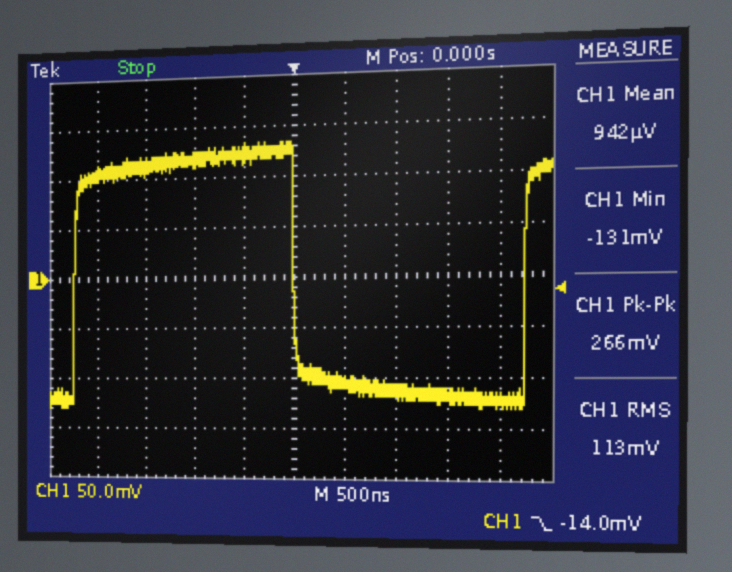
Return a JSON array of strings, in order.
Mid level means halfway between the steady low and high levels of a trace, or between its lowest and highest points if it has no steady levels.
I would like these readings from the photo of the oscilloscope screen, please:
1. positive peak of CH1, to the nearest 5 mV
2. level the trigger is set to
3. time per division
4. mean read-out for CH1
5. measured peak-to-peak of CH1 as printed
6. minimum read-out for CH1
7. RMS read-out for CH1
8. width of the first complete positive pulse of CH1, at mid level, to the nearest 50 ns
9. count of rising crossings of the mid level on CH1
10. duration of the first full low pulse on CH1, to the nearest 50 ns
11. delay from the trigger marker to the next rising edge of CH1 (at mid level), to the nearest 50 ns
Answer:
["135 mV", "-14.0 mV", "500 ns", "942 µV", "266 mV", "-131 mV", "113 mV", "2.25 µs", "2", "2.25 µs", "2.25 µs"]
